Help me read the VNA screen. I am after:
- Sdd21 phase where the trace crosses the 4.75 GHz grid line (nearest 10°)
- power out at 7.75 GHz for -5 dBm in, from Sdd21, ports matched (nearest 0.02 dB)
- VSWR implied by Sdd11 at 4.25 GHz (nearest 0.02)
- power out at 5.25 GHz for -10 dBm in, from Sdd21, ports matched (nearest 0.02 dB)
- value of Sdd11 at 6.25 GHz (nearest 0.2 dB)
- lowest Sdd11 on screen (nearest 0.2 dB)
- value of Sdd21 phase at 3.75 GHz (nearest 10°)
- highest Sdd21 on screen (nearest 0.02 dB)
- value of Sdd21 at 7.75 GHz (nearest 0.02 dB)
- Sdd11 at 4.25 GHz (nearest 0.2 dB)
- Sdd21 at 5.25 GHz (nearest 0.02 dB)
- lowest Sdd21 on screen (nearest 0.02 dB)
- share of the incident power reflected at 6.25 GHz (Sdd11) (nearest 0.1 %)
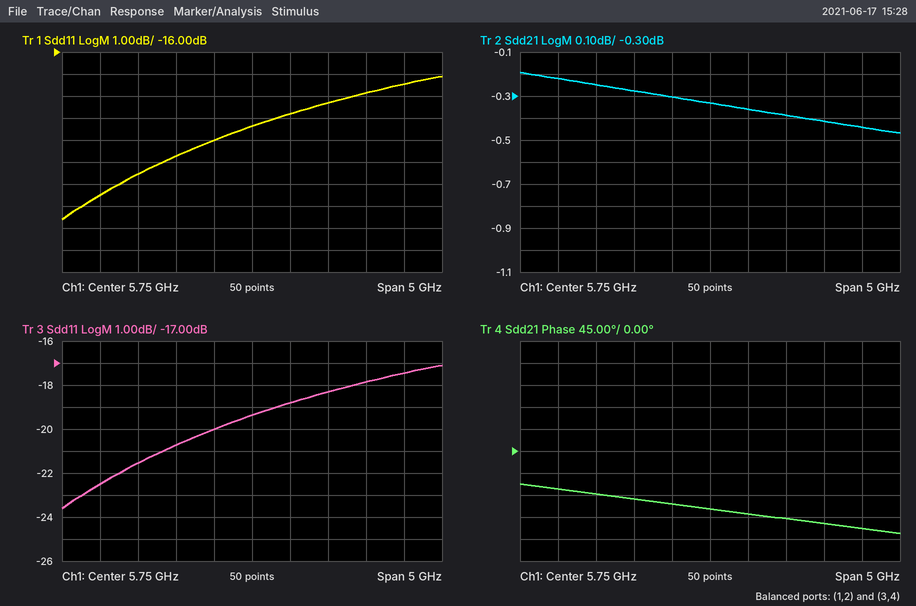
-100°
-5.44 dBm
1.18
-10.30 dBm
-18.8 dB
-23.6 dB
-80°
-0.20 dB
-0.44 dB
-21.6 dB
-0.30 dB
-0.46 dB
1.3 %
